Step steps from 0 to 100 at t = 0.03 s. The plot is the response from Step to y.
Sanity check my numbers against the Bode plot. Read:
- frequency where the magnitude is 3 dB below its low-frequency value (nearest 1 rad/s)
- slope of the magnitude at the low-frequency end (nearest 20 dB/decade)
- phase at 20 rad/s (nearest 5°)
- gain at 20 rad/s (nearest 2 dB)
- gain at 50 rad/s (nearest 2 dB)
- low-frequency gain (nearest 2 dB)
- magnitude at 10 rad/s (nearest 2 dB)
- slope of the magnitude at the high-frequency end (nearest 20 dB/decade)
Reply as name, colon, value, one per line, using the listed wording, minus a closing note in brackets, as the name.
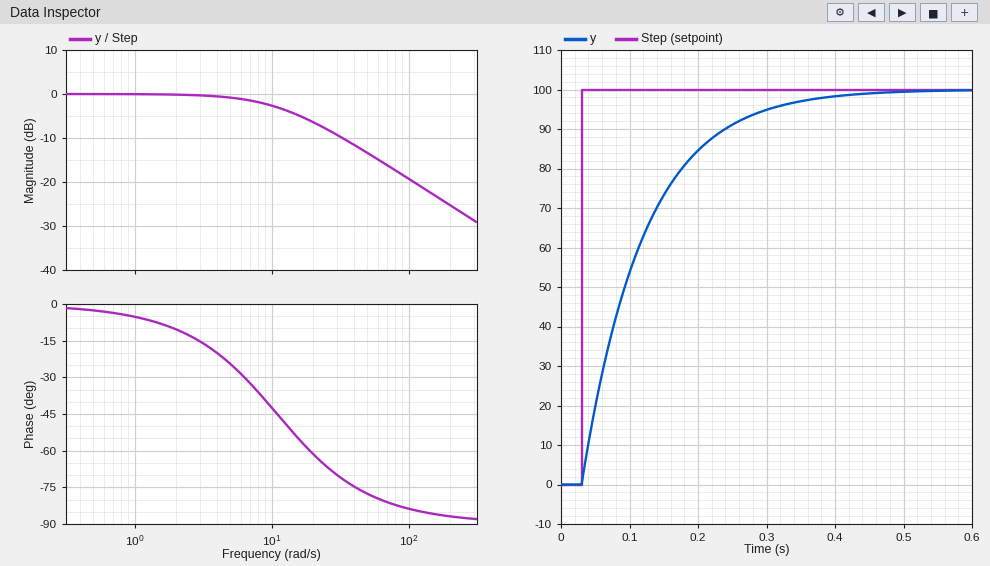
frequency where the magnitude is 3 dB below its low-frequency value: 11 rad/s
slope of the magnitude at the low-frequency end: 0 dB/decade
phase at 20 rad/s: -60°
gain at 20 rad/s: -6 dB
gain at 50 rad/s: -14 dB
low-frequency gain: 0 dB
magnitude at 10 rad/s: -2 dB
slope of the magnitude at the high-frequency end: -20 dB/decade
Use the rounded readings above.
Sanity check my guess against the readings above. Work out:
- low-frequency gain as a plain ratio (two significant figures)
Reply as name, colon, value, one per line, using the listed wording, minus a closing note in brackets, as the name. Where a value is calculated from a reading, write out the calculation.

low-frequency gain as a plain ratio: 10^(0 / 20) = 1.0
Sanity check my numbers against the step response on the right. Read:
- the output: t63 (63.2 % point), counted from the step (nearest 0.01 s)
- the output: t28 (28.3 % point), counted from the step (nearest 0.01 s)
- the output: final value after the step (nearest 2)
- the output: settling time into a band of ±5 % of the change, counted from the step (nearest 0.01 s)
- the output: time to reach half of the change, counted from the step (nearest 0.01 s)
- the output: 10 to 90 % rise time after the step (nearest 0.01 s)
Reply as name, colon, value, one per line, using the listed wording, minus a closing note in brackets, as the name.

the output: t63 (63.2 % point), counted from the step: 0.09 s
the output: t28 (28.3 % point), counted from the step: 0.03 s
the output: final value after the step: 100
the output: settling time into a band of ±5 % of the change, counted from the step: 0.27 s
the output: time to reach half of the change, counted from the step: 0.06 s
the output: 10 to 90 % rise time after the step: 0.20 s
